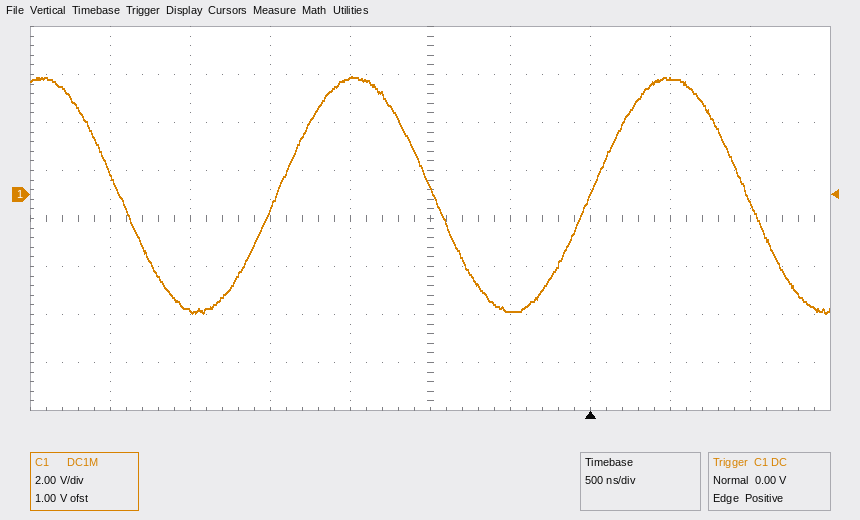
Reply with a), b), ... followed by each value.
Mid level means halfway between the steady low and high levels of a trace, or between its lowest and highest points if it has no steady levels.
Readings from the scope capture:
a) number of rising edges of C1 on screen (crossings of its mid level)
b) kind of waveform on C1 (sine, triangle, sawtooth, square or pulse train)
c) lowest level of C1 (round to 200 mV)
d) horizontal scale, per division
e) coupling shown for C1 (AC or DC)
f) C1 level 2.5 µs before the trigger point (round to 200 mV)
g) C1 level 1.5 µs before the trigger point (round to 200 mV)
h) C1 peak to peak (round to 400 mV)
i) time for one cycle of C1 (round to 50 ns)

a) 2
b) sine
c) -5.0 V
d) 500 ns
e) DC
f) -4.8 V
g) 4.8 V
h) 10.0 V
i) 1.95 µs
